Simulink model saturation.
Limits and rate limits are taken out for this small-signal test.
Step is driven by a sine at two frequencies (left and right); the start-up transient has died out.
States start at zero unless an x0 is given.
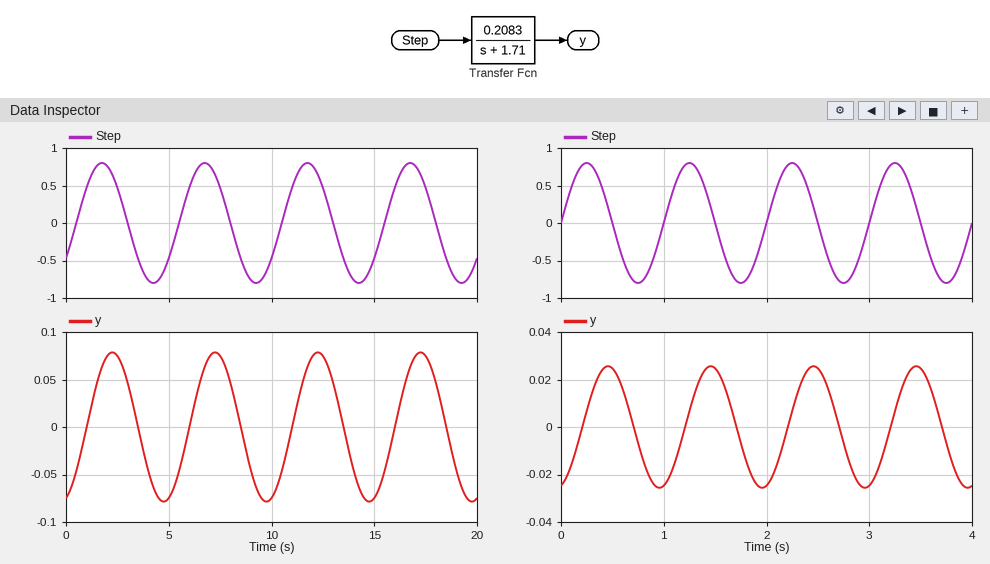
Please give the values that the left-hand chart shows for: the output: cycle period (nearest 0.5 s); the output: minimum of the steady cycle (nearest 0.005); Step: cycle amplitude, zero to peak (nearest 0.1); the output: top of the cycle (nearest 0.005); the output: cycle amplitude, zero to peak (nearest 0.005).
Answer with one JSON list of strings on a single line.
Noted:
["5.0 s", "-0.080", "0.8", "0.080", "0.080"]
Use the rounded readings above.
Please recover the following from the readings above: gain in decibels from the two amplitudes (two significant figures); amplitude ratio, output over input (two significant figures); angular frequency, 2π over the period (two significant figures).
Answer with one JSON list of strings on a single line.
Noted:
["-20 dB", "0.10", "1.3 rad/s"]
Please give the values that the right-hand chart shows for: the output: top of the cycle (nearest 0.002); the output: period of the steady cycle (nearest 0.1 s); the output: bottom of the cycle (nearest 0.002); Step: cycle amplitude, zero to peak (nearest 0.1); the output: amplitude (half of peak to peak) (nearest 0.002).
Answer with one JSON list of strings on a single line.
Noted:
["0.026", "1.0 s", "-0.026", "0.8", "0.026"]
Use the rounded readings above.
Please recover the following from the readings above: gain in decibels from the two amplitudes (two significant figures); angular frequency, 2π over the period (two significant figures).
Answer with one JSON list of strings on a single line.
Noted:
["-30 dB", "6.3 rad/s"]
